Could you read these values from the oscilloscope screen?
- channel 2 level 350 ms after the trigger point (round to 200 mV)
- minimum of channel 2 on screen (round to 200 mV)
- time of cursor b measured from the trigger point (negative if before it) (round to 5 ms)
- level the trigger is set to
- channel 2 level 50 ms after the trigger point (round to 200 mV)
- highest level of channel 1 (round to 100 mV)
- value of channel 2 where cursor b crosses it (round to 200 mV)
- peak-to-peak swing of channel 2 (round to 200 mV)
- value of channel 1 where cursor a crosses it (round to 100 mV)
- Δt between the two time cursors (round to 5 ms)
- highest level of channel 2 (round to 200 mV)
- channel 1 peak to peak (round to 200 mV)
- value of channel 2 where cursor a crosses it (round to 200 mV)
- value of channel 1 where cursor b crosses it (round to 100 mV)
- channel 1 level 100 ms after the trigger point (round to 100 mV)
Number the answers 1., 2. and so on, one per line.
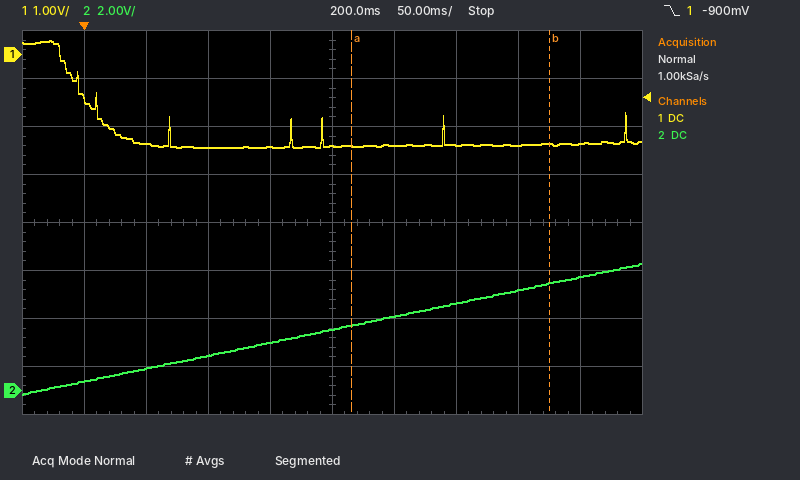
1. 4.2 V
2. -200 mV
3. +375 ms
4. -900 mV
5. 1.0 V
6. 300 mV
7. 4.4 V
8. 5.4 V
9. -1.9 V
10. 160 ms
11. 5.2 V
12. 2.2 V
13. 2.8 V
14. -1.9 V
15. -1.9 V
